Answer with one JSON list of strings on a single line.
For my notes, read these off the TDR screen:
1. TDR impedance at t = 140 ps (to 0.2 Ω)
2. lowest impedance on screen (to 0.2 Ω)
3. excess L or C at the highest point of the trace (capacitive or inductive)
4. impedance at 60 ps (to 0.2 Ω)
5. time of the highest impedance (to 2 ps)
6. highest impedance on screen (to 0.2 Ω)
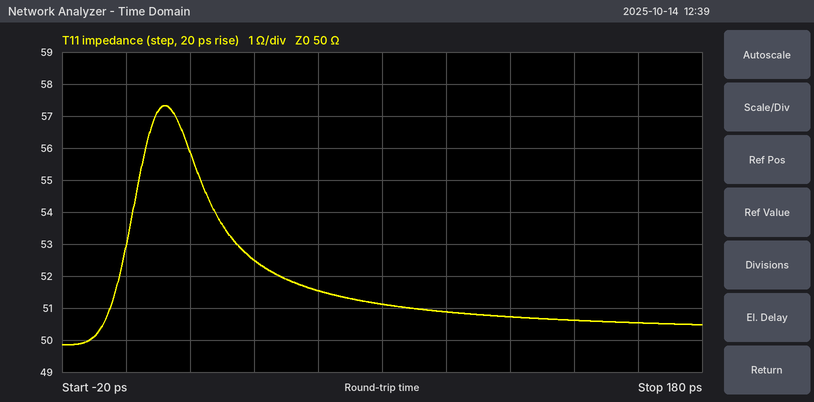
["50.6 Ω", "49.8 Ω", "inductive", "51.6 Ω", "12 ps", "57.4 Ω"]
